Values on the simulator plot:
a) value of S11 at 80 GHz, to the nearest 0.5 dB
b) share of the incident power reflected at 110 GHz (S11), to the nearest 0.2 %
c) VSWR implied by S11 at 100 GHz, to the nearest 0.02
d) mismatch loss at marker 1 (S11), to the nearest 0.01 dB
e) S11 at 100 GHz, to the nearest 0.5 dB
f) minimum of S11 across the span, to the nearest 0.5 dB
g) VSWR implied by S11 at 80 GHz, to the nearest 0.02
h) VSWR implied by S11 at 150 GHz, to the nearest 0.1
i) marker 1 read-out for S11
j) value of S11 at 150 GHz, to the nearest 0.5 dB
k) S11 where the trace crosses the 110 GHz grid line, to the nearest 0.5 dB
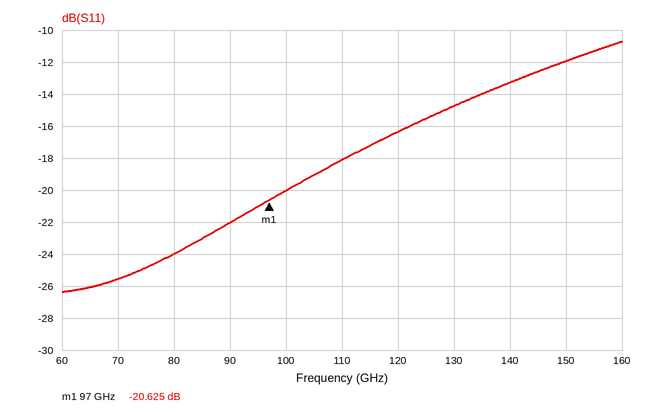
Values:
-24.0 dB
1.6 %
1.22
0.04 dB
-20.0 dB
-26.5 dB
1.14
1.7
-20.625 dB
-12.0 dB
-18.0 dB
